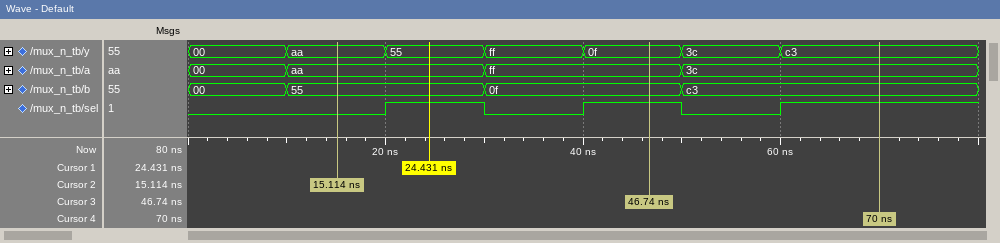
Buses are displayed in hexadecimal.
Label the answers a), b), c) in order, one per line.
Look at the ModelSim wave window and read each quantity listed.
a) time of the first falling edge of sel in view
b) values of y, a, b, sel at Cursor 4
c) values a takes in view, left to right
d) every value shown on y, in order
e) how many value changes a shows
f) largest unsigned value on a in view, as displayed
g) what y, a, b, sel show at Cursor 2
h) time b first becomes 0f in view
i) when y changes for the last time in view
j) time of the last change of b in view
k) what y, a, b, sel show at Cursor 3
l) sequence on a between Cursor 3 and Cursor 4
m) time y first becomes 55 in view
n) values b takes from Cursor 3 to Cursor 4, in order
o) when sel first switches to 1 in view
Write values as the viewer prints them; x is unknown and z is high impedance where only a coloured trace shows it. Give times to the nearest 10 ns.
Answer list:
a) 30 ns
b) y=c3, a=3c, b=c3, sel=1
c) 00, aa, ff, 3c
d) 00, aa, 55, ff, 0f, 3c, c3
e) 3
f) ff
g) y=aa, a=aa, b=55, sel=0
h) 30 ns
i) 60 ns
j) 50 ns
k) y=0f, a=ff, b=0f, sel=1
l) ff, 3c
m) 20 ns
n) 0f, c3
o) 20 ns
